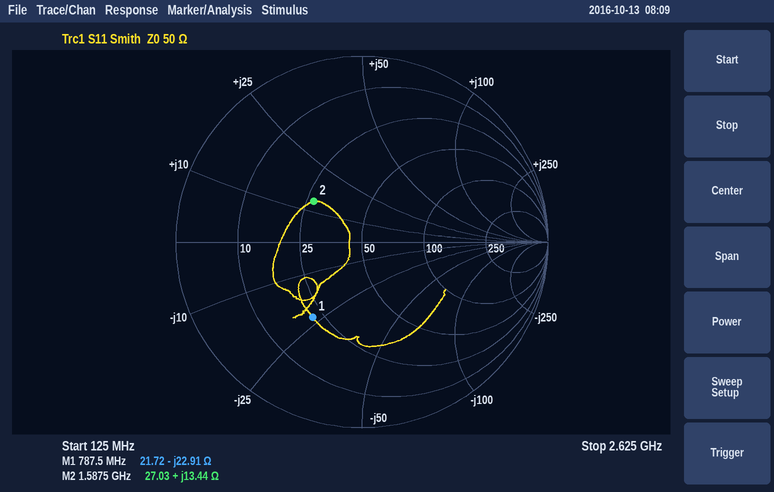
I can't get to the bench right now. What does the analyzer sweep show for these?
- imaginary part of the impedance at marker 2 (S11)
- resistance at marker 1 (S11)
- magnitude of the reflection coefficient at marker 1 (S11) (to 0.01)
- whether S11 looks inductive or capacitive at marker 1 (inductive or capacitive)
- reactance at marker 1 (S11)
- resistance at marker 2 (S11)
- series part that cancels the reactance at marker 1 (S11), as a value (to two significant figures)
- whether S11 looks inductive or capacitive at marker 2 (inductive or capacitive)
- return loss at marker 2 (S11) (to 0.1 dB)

+13.44 Ω
21.72 Ω
0.48
capacitive
-22.91 Ω
27.03 Ω
4.6 nH
inductive
9.4 dB
